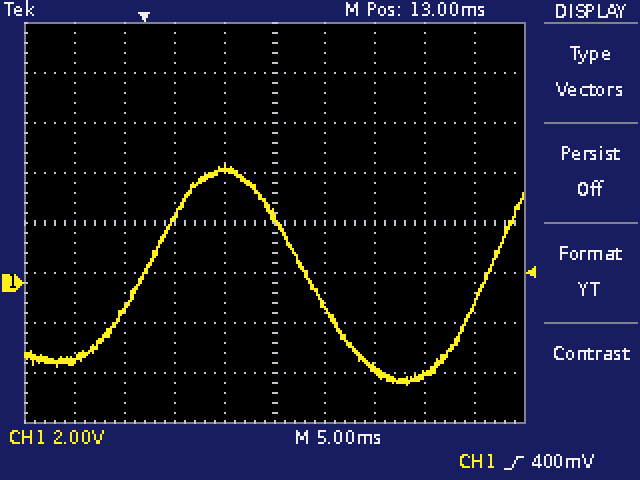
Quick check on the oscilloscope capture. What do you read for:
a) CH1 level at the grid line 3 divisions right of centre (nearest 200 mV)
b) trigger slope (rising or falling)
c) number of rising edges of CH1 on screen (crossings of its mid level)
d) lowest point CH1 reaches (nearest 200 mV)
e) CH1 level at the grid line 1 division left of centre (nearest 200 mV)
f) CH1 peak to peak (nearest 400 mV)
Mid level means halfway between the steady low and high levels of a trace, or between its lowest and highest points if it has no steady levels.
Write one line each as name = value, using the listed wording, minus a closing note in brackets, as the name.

CH1 level at the grid line 3 divisions right of centre = -3.6 V
trigger slope = rising
number of rising edges of CH1 on screen = 2
lowest point CH1 reaches = -4.0 V
CH1 level at the grid line 1 division left of centre = 4.6 V
CH1 peak to peak = 8.8 V
